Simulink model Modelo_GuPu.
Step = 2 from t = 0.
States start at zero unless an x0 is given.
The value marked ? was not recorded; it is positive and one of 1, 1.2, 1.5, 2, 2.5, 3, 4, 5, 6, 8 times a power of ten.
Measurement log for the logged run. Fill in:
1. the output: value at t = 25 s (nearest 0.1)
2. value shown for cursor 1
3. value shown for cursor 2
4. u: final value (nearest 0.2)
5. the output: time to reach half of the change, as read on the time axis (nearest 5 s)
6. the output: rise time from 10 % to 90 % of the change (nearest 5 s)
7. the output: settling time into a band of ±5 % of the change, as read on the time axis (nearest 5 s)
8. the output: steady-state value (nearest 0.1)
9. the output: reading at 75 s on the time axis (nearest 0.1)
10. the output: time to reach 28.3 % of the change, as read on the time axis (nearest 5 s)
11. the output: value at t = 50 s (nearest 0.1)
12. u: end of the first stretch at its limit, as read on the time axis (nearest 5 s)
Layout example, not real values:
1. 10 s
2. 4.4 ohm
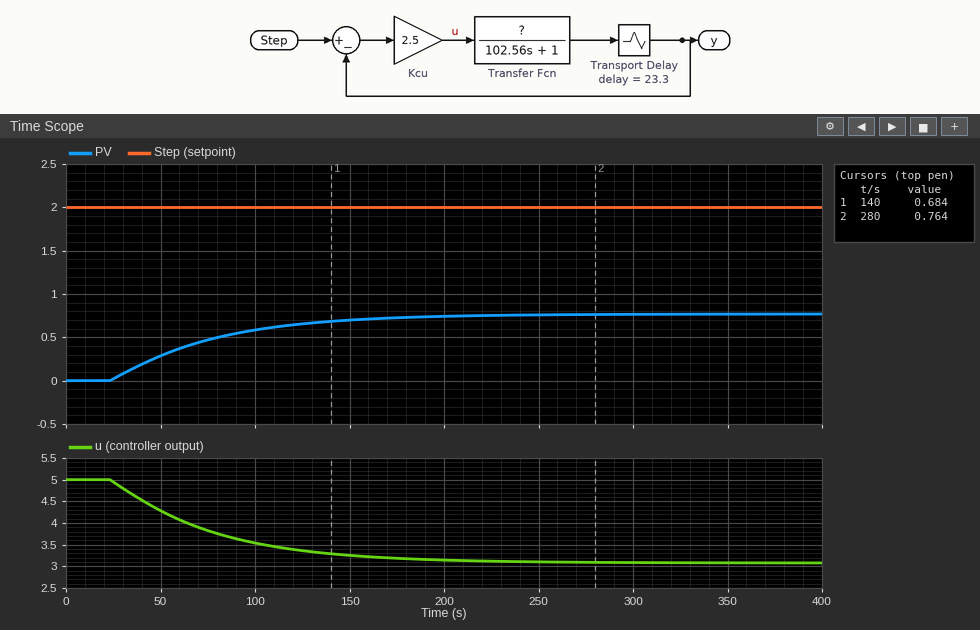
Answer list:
1. 0.0
2. 0.684
3. 0.764
4. 3.0
5. 60 s
6. 115 s
7. 180 s
8. 0.8
9. 0.5
10. 45 s
11. 0.3
12. 25 s
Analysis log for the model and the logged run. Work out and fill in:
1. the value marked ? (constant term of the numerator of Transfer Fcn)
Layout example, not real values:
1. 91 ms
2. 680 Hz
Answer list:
1. 0.25
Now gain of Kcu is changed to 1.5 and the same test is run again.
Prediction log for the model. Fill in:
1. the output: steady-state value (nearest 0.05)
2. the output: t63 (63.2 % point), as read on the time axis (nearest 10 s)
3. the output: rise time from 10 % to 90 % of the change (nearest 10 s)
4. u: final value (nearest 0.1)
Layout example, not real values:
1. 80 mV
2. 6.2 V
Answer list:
1. 0.55
2. 90 s
3. 150 s
4. 2.2
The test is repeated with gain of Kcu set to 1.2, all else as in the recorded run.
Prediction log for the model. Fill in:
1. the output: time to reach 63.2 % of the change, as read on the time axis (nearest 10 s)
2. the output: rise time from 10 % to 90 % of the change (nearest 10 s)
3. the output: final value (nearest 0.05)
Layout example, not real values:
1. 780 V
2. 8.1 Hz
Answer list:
1. 100 s
2. 160 s
3. 0.45
